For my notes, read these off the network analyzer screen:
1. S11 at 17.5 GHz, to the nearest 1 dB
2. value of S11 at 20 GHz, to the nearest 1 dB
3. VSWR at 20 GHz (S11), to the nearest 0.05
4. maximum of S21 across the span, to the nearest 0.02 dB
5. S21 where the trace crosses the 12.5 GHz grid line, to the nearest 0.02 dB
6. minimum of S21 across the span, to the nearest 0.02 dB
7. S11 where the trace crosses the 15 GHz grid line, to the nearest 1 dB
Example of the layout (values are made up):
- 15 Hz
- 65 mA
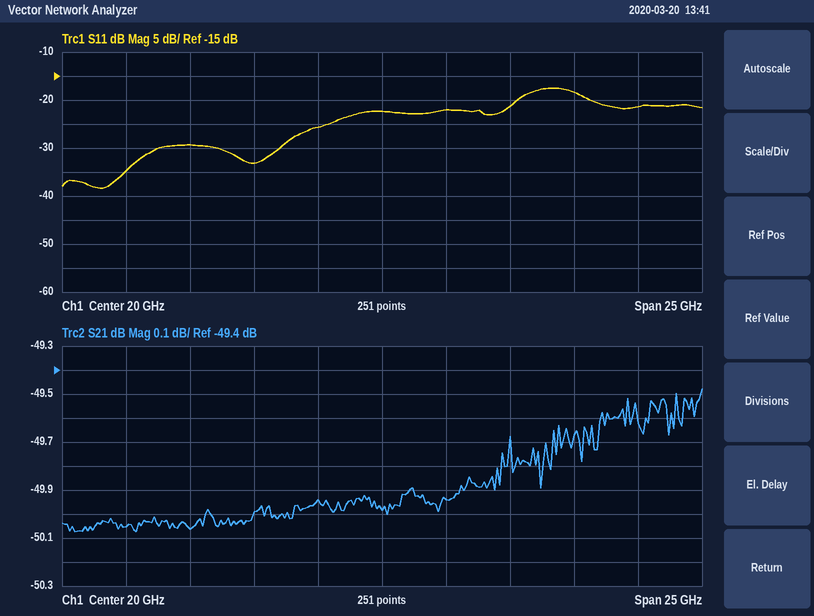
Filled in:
- -26 dB
- -22 dB
- 1.15
- -49.48 dB
- -50.06 dB
- -50.08 dB
- -33 dB
